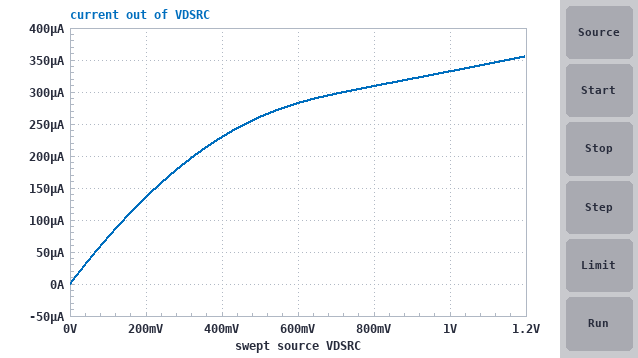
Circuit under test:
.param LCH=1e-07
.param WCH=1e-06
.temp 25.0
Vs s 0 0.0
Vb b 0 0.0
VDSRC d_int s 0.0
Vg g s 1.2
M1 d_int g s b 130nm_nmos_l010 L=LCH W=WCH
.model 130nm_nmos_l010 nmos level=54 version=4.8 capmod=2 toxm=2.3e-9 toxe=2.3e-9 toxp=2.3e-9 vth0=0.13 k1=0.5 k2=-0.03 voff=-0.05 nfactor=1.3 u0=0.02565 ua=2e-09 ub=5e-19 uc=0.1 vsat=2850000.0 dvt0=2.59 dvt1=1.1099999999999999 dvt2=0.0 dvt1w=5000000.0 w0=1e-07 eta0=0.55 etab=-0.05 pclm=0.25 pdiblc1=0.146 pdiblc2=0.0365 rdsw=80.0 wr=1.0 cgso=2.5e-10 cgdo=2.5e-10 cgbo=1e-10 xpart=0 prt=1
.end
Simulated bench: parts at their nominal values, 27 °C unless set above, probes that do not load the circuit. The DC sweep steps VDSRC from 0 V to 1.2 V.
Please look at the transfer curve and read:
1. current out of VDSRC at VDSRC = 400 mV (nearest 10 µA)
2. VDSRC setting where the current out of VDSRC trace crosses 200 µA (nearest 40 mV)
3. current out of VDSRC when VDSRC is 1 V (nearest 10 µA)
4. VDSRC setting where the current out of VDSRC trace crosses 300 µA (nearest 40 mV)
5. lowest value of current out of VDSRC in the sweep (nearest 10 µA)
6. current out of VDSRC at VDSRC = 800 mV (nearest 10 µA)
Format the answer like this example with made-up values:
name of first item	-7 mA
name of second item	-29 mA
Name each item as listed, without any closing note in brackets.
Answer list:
current out of VDSRC at VDSRC = 400 mV	230 µA
VDSRC setting where the current out of VDSRC trace crosses 200 µA	320 mV
current out of VDSRC when VDSRC is 1 V	330 µA
VDSRC setting where the current out of VDSRC trace crosses 300 µA	720 mV
lowest value of current out of VDSRC in the sweep	0 A
current out of VDSRC at VDSRC = 800 mV	310 µA
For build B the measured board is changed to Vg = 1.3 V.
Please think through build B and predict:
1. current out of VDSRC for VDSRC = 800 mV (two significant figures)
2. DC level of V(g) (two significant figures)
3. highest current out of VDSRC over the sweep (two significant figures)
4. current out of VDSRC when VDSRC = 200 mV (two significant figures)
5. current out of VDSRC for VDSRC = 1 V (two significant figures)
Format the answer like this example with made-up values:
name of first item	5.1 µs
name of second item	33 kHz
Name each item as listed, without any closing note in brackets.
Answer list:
current out of VDSRC for VDSRC = 800 mV	380 µA
DC level of V(g)	1.3 V
highest current out of VDSRC over the sweep	430 µA
current out of VDSRC when VDSRC = 200 mV	150 µA
current out of VDSRC for VDSRC = 1 V	400 µA
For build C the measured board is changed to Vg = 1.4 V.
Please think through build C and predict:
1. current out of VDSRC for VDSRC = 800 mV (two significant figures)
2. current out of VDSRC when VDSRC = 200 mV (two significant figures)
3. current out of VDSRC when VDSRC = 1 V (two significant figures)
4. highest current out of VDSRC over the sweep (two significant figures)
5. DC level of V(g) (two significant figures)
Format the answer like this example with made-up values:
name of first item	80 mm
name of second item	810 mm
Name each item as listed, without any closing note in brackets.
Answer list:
current out of VDSRC for VDSRC = 800 mV	450 µA
current out of VDSRC when VDSRC = 200 mV	170 µA
current out of VDSRC when VDSRC = 1 V	480 µA
highest current out of VDSRC over the sweep	510 µA
DC level of V(g)	1.4 V
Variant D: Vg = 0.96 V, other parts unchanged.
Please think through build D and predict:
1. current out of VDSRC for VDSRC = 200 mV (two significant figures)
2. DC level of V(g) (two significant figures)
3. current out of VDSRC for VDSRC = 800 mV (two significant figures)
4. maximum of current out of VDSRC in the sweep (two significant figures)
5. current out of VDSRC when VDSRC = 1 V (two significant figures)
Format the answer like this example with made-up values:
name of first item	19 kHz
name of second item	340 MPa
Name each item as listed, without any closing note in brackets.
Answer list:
current out of VDSRC for VDSRC = 200 mV	86 µA
DC level of V(g)	960 mV
current out of VDSRC for VDSRC = 800 mV	160 µA
maximum of current out of VDSRC in the sweep	200 µA
current out of VDSRC when VDSRC = 1 V	180 µA
